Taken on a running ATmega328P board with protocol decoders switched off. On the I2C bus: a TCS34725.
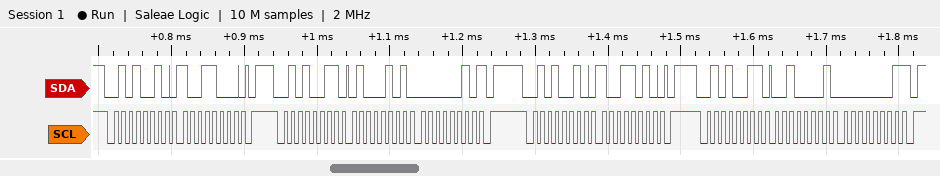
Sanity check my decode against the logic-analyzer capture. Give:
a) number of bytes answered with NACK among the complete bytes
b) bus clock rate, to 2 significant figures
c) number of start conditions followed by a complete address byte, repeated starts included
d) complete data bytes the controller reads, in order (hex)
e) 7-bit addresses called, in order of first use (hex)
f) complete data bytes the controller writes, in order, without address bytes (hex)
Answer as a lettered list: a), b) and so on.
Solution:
a) 2
b) 100 kHz
c) 4
d) 45 02 21 01
e) 0x29
f) 98 9A
